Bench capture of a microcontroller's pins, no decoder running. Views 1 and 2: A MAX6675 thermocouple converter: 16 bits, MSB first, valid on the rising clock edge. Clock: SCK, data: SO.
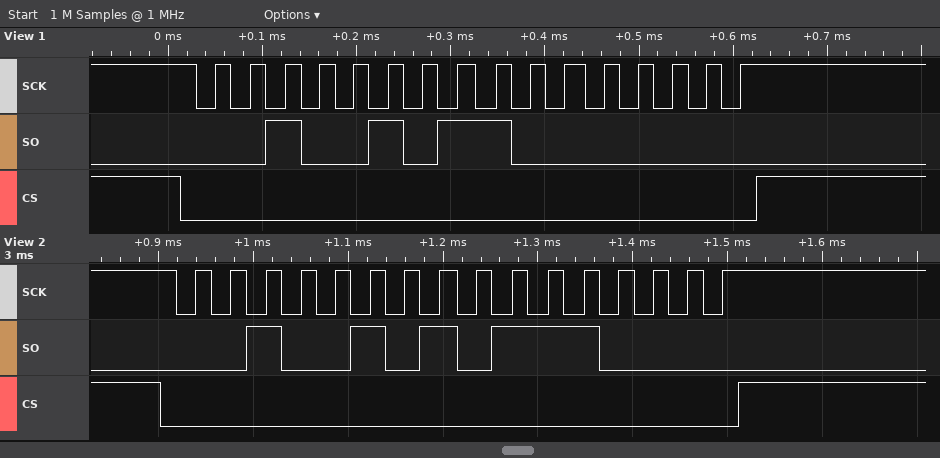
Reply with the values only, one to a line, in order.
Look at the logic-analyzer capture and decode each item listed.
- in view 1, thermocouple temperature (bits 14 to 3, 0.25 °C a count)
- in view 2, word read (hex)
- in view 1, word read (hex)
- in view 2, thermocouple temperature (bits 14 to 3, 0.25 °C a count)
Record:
300.00 °C
0x2570
0x2580
299.50 °C
